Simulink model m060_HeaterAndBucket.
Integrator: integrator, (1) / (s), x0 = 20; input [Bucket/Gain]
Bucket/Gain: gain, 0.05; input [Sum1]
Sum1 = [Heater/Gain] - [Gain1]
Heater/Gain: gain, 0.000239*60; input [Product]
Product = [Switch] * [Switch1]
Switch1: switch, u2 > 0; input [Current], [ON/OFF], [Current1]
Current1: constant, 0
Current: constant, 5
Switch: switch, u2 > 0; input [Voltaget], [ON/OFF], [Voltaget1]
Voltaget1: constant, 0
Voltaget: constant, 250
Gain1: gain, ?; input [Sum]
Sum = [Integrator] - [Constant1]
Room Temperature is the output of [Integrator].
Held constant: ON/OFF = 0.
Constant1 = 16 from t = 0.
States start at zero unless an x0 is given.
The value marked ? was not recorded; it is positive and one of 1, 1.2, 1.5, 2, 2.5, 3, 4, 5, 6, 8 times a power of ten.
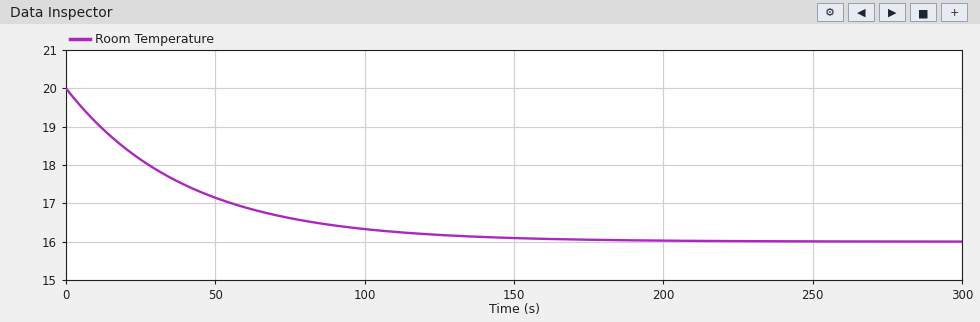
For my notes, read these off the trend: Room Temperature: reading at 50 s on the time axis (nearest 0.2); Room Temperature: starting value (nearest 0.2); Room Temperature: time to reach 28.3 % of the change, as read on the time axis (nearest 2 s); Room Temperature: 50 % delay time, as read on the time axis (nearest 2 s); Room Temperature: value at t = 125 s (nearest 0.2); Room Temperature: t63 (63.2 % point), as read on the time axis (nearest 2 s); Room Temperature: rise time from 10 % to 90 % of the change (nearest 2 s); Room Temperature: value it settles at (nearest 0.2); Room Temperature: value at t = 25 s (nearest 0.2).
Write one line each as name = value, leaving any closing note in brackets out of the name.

Room Temperature: reading at 50 s on the time axis = 17.2
Room Temperature: starting value = 20.0
Room Temperature: time to reach 28.3 % of the change, as read on the time axis = 14 s
Room Temperature: 50 % delay time, as read on the time axis = 28 s
Room Temperature: value at t = 125 s = 16.2
Room Temperature: t63 (63.2 % point), as read on the time axis = 40 s
Room Temperature: rise time from 10 % to 90 % of the change = 88 s
Room Temperature: value it settles at = 16.0
Room Temperature: value at t = 25 s = 18.2
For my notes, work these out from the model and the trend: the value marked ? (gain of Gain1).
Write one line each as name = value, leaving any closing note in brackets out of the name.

the value marked ? = 0.5
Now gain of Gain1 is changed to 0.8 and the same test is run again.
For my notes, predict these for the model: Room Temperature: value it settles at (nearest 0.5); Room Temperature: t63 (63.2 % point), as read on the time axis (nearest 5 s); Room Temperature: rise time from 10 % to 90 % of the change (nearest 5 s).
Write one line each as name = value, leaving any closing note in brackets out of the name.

Room Temperature: value it settles at = 16.0
Room Temperature: t63 (63.2 % point), as read on the time axis = 25 s
Room Temperature: rise time from 10 % to 90 % of the change = 55 s
